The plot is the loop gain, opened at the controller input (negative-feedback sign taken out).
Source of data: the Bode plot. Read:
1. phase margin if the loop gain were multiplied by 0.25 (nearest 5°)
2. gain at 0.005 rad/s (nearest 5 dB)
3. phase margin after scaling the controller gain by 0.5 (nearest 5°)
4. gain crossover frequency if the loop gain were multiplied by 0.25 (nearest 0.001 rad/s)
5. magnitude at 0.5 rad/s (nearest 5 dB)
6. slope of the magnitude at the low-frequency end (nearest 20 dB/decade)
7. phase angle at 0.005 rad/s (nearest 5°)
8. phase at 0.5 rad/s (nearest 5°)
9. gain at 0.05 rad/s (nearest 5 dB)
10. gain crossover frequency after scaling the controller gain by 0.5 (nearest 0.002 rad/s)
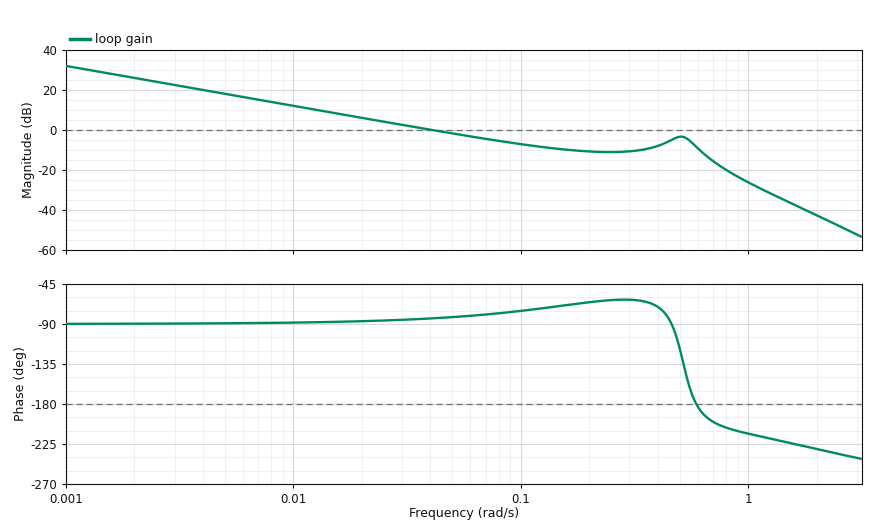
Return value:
90°
20 dB
95°
0.010 rad/s
-5 dB
-20 dB/decade
-90°
-120°
0 dB
0.020 rad/s
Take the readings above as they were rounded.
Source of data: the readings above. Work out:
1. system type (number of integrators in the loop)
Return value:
1
